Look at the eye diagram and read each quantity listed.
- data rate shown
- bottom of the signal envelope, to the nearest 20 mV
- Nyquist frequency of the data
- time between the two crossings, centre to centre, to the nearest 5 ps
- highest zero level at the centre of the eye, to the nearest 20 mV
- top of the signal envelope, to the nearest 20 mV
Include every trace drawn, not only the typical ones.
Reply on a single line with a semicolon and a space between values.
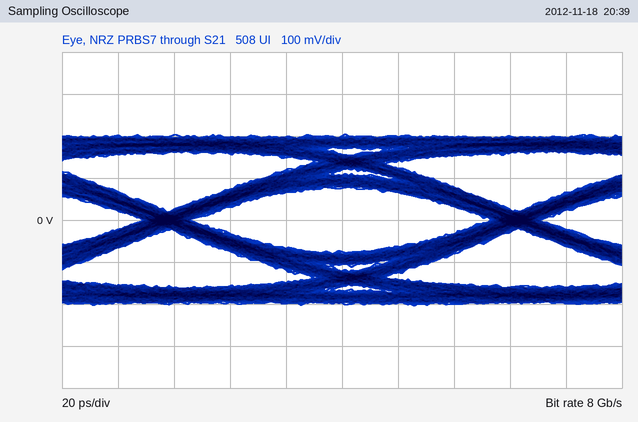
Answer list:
8 Gb/s; -200 mV; 4 GHz; 125 ps; -80 mV; 200 mV
